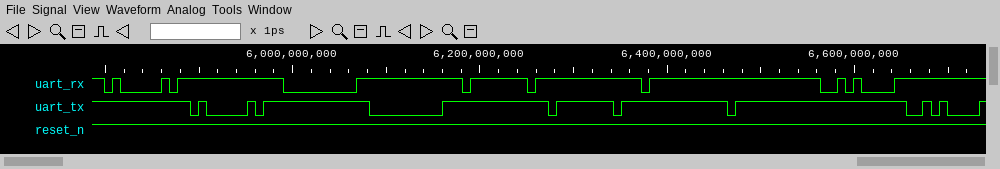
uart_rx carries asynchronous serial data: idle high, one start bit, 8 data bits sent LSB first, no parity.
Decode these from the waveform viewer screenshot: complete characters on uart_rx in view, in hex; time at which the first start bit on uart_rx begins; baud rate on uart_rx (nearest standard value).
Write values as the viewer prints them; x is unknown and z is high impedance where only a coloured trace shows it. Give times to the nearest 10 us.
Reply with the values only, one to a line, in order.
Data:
41, 00, 7F, FF, 0A
5800 us
115200 baud
